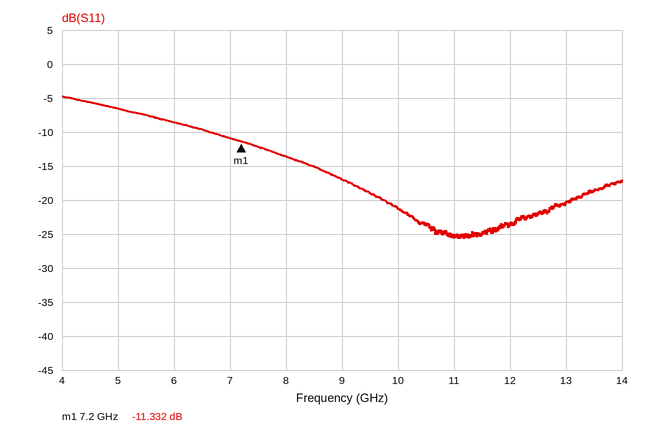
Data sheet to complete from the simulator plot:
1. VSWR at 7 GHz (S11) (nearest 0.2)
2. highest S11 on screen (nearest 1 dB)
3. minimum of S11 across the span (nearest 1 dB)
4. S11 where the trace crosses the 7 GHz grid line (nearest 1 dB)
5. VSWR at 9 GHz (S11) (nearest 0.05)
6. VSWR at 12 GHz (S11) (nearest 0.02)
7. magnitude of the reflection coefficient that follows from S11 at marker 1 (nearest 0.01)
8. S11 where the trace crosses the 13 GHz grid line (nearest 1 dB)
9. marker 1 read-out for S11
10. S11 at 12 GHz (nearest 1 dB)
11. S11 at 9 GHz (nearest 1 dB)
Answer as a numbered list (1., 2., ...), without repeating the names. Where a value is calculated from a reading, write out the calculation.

1. |Γ| = 10^(-11/20) = 0.2818; VSWR = (1 + 0.2818)/(1 − 0.2818) ≈ 1.8
2. -5 dB
3. -26 dB
4. -11 dB
5. |Γ| = 10^(-17/20) = 0.1413; VSWR = (1 + 0.1413)/(1 − 0.1413) ≈ 1.33, so 1.35 to the nearest 0.05
6. |Γ| = 10^(-24/20) = 0.0631; VSWR = (1 + 0.0631)/(1 − 0.0631) ≈ 1.13, so 1.14 to the nearest 0.02
7. 10^(-11.332/20) ≈ 0.27
8. -20 dB
9. -11.332 dB
10. -24 dB
11. -17 dB
